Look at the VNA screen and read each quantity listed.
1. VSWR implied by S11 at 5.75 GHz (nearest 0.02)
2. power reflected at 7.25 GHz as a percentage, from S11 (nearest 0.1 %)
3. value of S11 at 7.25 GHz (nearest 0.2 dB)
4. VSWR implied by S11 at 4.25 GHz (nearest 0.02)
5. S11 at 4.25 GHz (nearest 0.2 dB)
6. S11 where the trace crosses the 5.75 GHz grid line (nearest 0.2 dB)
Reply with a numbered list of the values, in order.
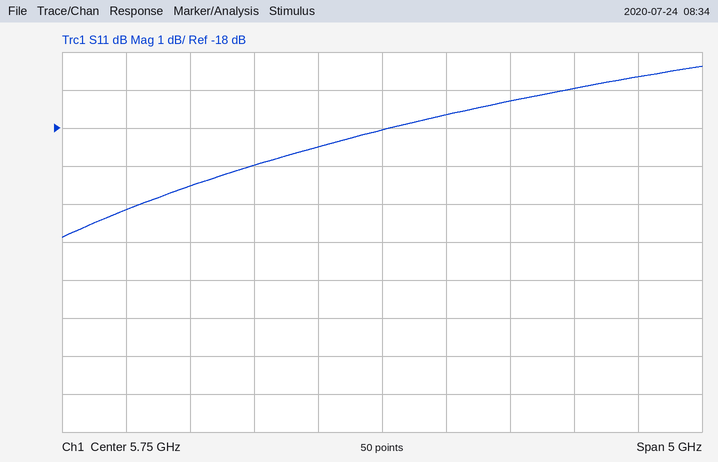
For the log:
1. 1.28
2. 2.0 %
3. -17.0 dB
4. 1.24
5. -19.6 dB
6. -18.0 dB
